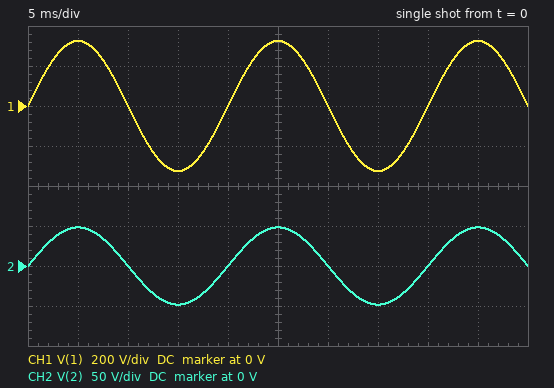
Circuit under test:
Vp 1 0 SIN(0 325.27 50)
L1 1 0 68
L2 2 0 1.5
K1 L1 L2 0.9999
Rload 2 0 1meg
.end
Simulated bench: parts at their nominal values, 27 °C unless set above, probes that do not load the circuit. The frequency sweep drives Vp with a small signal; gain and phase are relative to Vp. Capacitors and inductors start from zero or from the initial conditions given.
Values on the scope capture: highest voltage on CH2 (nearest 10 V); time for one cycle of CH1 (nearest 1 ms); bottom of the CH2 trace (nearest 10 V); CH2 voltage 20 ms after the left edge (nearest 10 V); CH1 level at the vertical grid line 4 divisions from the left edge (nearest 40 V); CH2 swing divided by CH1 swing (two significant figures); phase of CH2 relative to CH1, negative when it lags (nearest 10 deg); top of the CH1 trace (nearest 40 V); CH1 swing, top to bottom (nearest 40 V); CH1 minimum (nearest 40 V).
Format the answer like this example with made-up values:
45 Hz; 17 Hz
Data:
50 V; 20 ms; -50 V; 0 V; 0 V; 0.15; 0 deg; 320 V; 640 V; -320 V
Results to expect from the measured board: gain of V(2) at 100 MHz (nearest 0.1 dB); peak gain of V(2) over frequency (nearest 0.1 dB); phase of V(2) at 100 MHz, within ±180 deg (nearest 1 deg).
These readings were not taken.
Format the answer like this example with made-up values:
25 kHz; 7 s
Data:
-16.7 dB; -16.6 dB; -11 deg
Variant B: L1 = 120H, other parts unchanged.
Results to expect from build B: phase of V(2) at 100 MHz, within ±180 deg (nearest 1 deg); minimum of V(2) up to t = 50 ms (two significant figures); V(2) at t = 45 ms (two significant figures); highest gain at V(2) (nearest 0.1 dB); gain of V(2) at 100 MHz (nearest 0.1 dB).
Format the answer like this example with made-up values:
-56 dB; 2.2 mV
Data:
-11 deg; -36 V; 36 V; -19.0 dB; -19.2 dB
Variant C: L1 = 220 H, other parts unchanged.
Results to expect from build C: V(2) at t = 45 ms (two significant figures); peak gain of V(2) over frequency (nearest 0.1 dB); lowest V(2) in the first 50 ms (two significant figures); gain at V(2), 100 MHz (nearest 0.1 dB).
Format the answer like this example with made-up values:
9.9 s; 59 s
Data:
27 V; -21.7 dB; -27 V; -21.8 dB
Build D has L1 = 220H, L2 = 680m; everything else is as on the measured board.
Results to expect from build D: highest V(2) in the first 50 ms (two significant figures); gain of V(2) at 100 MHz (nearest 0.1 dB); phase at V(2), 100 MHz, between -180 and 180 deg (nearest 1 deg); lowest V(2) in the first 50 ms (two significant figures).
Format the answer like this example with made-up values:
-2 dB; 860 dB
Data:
18 V; -25.1 dB; -5 deg; -18 V
